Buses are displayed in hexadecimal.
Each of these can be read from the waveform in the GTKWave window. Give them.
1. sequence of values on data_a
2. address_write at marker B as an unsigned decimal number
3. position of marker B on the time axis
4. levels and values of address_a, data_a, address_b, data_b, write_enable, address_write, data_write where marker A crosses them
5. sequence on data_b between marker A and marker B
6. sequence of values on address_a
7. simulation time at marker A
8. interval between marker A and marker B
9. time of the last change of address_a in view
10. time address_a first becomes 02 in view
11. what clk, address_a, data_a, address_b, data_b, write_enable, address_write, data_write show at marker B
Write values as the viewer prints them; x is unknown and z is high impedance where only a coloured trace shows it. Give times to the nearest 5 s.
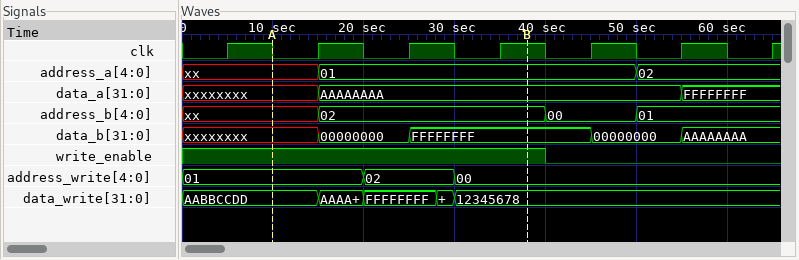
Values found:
xxxxxxxx, AAAAAAAA, FFFFFFFF
0
40 s
address_a=xx, data_a=xxxxxxxx, address_b=xx, data_b=xxxxxxxx, write_enable=1, address_write=01, data_write=AABBCCDD
xxxxxxxx, 00000000, FFFFFFFF
xx, 01, 02
10 s
30 s
50 s
50 s
clk=1, address_a=01, data_a=AAAAAAAA, address_b=02, data_b=FFFFFFFF, write_enable=1, address_write=00, data_write=12345678
